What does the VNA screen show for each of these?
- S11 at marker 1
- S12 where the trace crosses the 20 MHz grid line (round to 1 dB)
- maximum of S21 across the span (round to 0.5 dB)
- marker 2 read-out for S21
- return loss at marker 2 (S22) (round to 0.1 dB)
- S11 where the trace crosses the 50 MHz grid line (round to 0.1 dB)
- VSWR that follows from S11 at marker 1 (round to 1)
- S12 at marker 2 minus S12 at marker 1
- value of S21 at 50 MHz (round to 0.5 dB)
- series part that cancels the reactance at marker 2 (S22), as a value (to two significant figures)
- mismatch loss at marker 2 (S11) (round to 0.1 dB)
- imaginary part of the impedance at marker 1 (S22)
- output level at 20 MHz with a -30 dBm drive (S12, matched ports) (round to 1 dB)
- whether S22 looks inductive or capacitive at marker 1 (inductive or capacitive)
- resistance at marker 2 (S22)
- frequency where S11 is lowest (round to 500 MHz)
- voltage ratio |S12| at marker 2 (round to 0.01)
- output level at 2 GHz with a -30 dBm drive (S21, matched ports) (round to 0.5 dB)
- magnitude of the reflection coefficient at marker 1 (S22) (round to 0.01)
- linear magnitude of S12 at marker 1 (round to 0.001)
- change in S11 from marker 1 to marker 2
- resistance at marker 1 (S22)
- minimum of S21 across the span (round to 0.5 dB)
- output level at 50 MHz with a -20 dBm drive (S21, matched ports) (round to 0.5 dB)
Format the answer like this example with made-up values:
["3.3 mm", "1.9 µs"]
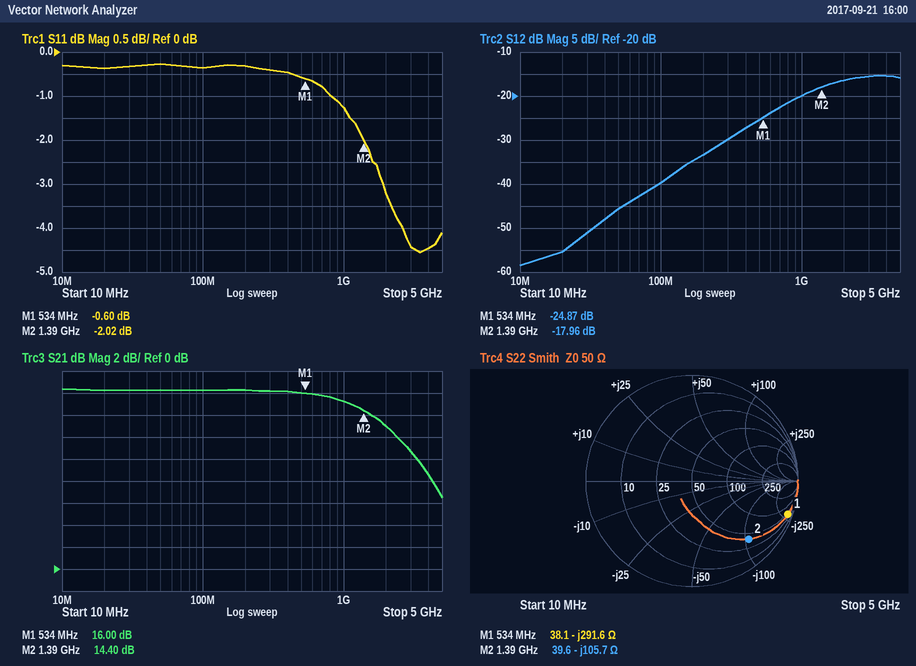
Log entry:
["-0.60 dB", "-55 dB", "16.5 dB", "14.40 dB", "2.3 dB", "-0.3 dB", "29", "6.91 dB", "16.5 dB", "12 nH", "4.3 dB", "-291.6 Ω", "-85 dBm", "capacitive", "39.6 Ω", "3.5 GHz", "0.13", "-17.0 dBm", "0.96", "0.057", "-1.42 dB", "38.1 Ω", "6.5 dB", "-3.5 dBm"]
